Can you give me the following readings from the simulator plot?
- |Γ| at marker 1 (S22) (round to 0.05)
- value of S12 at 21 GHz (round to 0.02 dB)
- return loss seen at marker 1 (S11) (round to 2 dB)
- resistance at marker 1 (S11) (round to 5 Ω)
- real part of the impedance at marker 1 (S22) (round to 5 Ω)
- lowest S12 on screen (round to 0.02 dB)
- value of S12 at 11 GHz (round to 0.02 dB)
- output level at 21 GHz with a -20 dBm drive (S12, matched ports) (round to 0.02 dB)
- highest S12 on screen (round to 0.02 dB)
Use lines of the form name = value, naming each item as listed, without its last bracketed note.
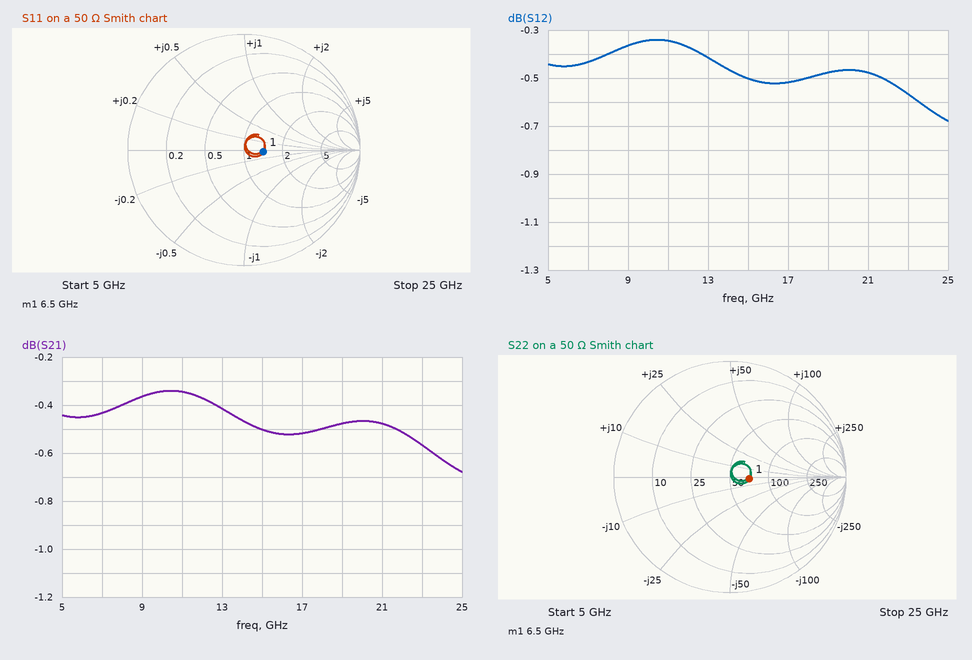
|Γ| at marker 1 (S22) = 0.15
value of S12 at 21 GHz = -0.48 dB
return loss seen at marker 1 (S11) = 16 dB
resistance at marker 1 (S11) = 70 Ω
real part of the impedance at marker 1 (S22) = 70 Ω
lowest S12 on screen = -0.68 dB
value of S12 at 11 GHz = -0.34 dB
output level at 21 GHz with a -20 dBm drive (S12, matched ports) = -20.48 dBm
highest S12 on screen = -0.34 dB
